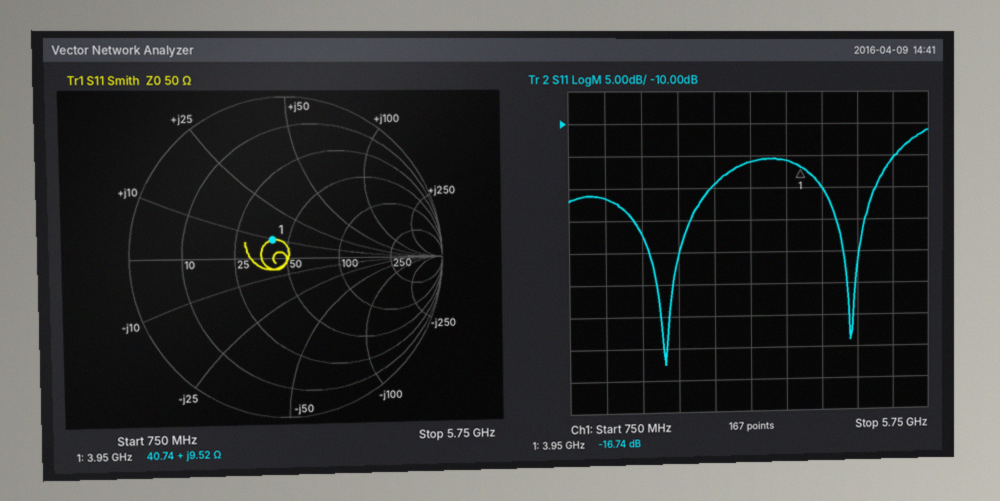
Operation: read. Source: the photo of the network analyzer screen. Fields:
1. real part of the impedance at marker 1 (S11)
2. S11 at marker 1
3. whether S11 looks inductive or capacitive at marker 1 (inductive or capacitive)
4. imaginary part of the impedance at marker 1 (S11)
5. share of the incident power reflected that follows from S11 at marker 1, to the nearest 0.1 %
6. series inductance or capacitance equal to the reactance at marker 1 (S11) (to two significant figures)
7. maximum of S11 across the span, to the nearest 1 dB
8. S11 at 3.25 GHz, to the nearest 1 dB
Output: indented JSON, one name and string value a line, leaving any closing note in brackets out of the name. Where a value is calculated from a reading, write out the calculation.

{
  "real part of the impedance at marker 1": "40.74 Ω",
  "S11 at marker 1": "-16.74 dB",
  "whether S11 looks inductive or capacitive at marker 1": "inductive",
  "imaginary part of the impedance at marker 1": "+9.52 Ω",
  "share of the incident power reflected that follows from S11 at marker 1, to the nearest 0.1 %": "10^(-16.74/10) ≈ 2.1 %",
  "series inductance or capacitance equal to the reactance at marker 1 (S11)": "L = 9.52 Ω/(2π × 3.95 GHz) ≈ 384 pH, so 380 pH to two significant figures",
  "maximum of S11 across the span, to the nearest 1 dB": "-11 dB",
  "S11 at 3.25 GHz, to the nearest 1 dB": "-16 dB"
}
